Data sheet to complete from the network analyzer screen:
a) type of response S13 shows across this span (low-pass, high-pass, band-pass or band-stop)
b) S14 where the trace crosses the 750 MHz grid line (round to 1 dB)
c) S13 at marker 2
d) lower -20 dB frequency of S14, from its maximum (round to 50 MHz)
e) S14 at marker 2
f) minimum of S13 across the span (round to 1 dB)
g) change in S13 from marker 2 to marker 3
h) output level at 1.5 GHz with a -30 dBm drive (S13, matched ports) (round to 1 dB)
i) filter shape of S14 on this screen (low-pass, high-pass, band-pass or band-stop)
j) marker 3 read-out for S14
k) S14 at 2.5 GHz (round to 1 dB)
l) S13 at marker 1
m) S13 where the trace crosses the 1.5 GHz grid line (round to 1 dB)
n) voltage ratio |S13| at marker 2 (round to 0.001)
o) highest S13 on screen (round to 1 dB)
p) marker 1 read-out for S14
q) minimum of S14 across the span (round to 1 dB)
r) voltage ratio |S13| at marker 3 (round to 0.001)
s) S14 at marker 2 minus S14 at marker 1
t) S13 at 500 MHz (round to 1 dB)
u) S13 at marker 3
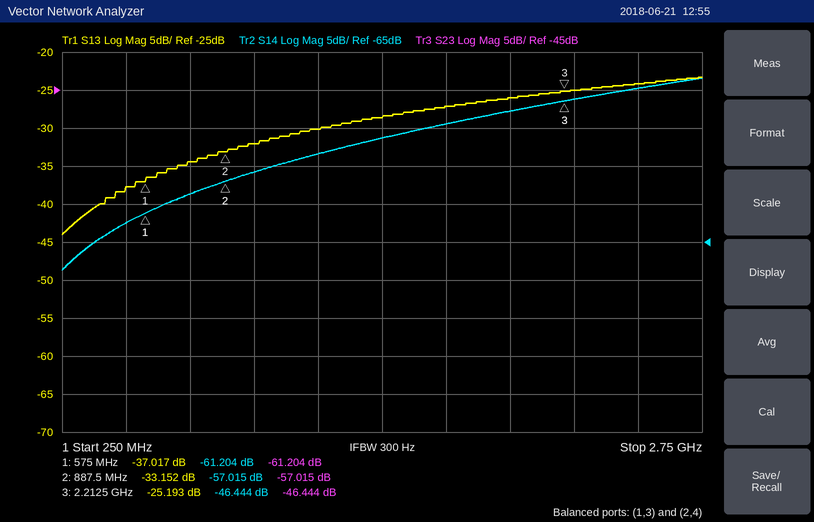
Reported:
high-pass
-59 dB
-33.152 dB
450 MHz
-57.015 dB
-44 dB
7.959 dB
-59 dBm
high-pass
-46.444 dB
-45 dB
-37.017 dB
-29 dB
0.022
-23 dB
-61.204 dB
-69 dB
0.055
4.189 dB
-38 dB
-25.193 dB
